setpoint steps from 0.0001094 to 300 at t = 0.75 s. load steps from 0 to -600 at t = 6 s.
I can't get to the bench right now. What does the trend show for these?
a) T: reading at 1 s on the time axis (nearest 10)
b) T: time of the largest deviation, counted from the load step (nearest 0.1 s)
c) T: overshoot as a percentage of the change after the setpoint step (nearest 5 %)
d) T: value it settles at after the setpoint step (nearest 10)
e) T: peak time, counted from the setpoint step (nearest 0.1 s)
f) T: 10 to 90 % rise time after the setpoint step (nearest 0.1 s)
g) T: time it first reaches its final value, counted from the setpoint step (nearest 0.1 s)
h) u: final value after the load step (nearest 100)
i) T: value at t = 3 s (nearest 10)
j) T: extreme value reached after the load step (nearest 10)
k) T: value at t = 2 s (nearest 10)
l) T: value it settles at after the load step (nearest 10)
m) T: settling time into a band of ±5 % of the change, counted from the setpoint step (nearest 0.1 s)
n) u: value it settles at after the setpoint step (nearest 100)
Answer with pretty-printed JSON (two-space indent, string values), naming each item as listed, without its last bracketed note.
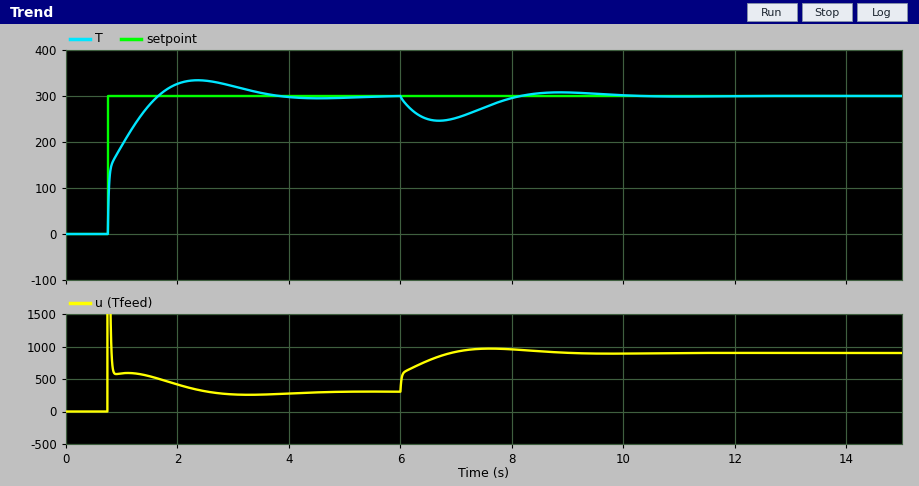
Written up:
{
  "T: reading at 1 s on the time axis": "190",
  "T: time of the largest deviation, counted from the load step": "0.7 s",
  "T: overshoot as a percentage of the change after the setpoint step": "10 %",
  "T: value it settles at after the setpoint step": "300",
  "T: peak time, counted from the setpoint step": "1.6 s",
  "T: 10 to 90 % rise time after the setpoint step": "0.7 s",
  "T: time it first reaches its final value, counted from the setpoint step": "0.9 s",
  "u: final value after the load step": "900",
  "T: value at t = 3 s": "320",
  "T: extreme value reached after the load step": "250",
  "T: value at t = 2 s": "330",
  "T: value it settles at after the load step": "300",
  "T: settling time into a band of ±5 % of the change, counted from the setpoint step": "2.5 s",
  "u: value it settles at after the setpoint step": "300"
}
